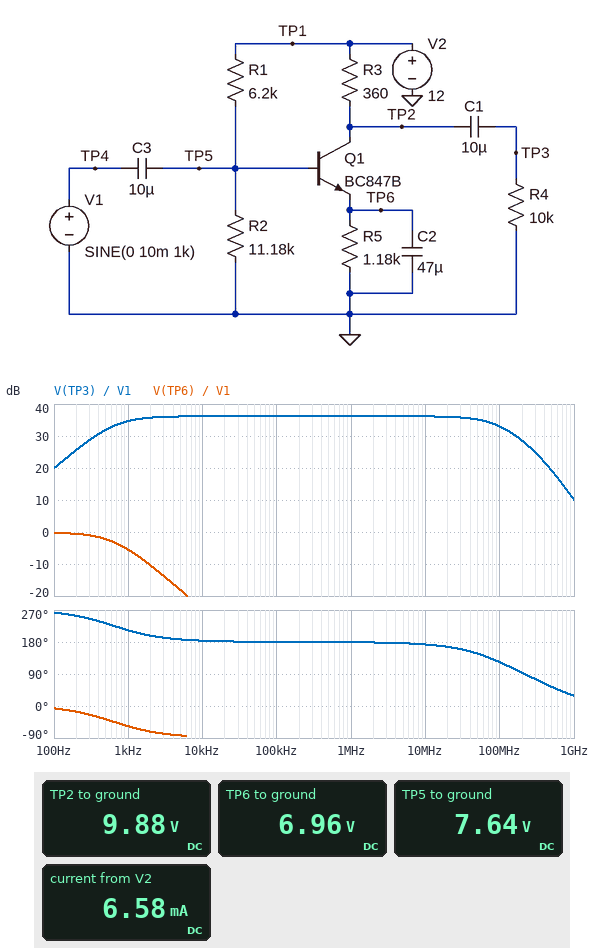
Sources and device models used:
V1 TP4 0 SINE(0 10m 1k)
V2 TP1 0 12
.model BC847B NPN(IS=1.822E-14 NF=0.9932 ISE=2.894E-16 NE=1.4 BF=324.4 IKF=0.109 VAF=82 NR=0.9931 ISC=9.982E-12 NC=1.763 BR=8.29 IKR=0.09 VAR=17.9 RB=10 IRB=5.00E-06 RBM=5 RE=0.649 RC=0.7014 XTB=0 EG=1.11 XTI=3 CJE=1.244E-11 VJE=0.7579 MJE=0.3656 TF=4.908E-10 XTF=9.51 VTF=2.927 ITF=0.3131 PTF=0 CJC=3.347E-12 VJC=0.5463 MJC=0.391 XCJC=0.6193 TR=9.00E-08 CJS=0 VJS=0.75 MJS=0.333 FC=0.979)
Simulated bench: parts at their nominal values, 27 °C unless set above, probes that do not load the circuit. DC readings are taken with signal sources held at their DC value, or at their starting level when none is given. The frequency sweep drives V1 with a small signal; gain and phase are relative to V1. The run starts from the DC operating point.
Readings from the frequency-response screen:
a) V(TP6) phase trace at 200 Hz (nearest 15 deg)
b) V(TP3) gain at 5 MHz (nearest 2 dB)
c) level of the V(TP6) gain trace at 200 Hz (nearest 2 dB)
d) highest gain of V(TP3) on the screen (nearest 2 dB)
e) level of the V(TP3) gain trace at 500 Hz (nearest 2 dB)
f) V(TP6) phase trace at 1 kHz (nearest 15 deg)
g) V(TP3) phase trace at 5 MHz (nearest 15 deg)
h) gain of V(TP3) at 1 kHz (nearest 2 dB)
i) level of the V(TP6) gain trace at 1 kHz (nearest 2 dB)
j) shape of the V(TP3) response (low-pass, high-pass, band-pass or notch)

-15 deg
36 dB
0 dB
36 dB
32 dB
-60 deg
180 deg
34 dB
-6 dB
band-pass
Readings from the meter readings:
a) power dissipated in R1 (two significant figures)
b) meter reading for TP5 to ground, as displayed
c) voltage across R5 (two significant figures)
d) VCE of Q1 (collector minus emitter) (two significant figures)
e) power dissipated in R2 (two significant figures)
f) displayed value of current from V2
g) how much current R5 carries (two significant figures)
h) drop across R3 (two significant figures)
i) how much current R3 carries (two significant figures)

3.1 mW
7.64 V
7.0 V
2.9 V
5.2 mW
6.58 mA
5.9 mA
2.1 V
5.9 mA
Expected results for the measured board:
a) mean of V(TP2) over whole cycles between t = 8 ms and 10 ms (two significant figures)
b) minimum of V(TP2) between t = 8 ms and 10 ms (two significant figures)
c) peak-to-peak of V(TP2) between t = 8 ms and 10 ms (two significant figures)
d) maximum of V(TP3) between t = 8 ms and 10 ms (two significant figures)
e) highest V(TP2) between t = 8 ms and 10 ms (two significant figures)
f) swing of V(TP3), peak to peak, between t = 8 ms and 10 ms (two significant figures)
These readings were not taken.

9.9 V
9.3 V
1.1 V
510 mV
10 V
1.1 V
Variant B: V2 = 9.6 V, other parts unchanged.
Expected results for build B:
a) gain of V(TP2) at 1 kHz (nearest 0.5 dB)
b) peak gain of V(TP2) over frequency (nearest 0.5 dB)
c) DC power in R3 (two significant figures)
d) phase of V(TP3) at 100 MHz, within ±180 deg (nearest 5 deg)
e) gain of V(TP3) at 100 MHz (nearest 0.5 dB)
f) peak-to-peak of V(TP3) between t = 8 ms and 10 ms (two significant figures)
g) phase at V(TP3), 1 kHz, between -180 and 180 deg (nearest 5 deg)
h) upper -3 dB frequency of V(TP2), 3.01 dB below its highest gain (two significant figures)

33.5 dB
34.5 dB
7.6 mW
125 deg
31.5 dB
920 mV
-150 deg
100 MHz
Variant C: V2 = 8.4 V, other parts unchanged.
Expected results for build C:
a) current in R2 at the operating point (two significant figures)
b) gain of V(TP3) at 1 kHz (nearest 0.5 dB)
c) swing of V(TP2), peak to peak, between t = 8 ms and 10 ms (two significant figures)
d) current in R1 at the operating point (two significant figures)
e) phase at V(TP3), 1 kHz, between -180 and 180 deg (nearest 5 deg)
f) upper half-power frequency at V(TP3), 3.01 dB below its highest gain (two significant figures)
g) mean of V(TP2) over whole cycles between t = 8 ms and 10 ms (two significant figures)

480 µA
32.5 dB
830 mV
490 µA
-155 deg
110 MHz
7.0 V
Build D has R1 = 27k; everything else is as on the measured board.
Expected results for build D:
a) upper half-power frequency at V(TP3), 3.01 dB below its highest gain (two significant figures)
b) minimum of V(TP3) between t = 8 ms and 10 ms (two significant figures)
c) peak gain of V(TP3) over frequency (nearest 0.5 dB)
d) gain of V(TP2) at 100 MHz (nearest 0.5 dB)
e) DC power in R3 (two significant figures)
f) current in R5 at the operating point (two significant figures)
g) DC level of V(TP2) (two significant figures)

180 MHz
-300 mV
29.5 dB
28.0 dB
2.0 mW
2.4 mA
11 V
